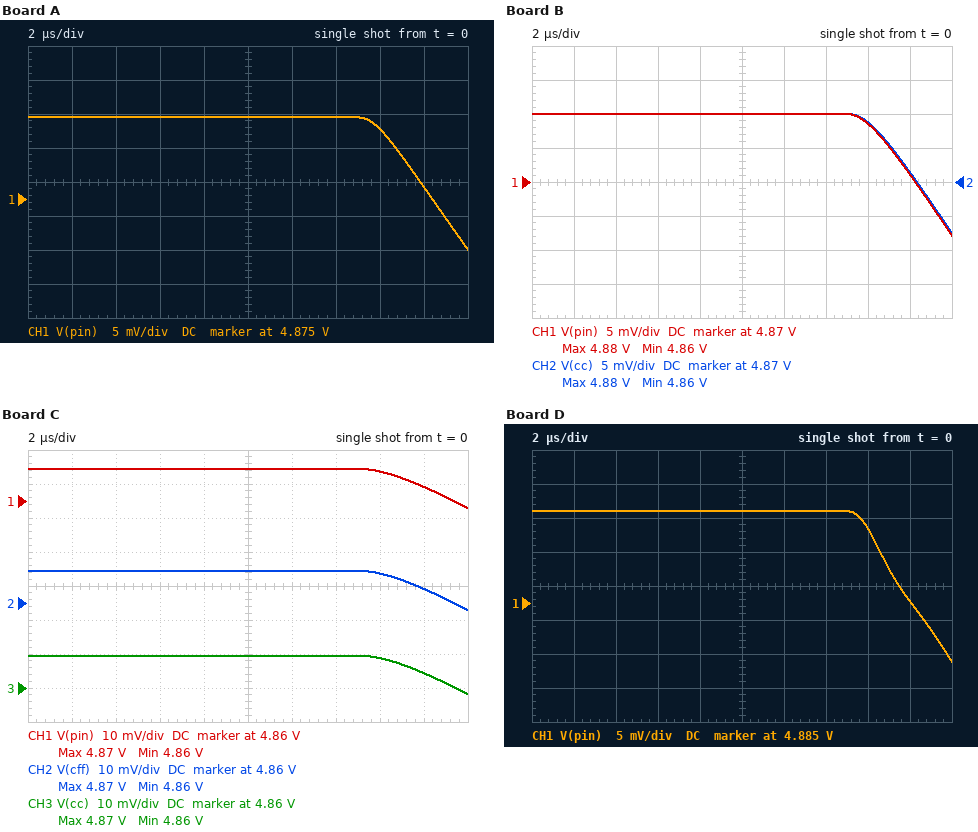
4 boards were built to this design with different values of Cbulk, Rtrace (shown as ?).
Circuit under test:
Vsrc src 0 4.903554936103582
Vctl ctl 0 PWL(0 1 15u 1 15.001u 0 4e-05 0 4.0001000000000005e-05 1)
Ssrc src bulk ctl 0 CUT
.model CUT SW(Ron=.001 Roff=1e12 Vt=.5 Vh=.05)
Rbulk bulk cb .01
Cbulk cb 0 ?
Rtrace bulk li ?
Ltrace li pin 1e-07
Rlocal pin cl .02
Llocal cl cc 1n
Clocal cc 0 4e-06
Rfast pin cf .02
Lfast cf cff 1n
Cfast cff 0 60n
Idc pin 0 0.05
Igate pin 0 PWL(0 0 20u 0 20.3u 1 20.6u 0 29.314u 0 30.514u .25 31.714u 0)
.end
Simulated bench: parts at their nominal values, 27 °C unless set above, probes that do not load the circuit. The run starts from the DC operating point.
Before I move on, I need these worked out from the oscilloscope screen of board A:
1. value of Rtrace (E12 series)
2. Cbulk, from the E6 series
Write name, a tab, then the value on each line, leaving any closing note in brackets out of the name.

value of Rtrace	0.33 Ω
Cbulk, from the E6 series	6.8 µF
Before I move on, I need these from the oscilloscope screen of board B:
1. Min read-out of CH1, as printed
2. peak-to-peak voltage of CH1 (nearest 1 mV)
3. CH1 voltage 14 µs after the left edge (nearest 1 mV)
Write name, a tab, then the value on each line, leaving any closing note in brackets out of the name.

Min read-out of CH1, as printed	4.86 V
peak-to-peak voltage of CH1	18 mV
CH1 voltage 14 µs after the left edge	4.880 V
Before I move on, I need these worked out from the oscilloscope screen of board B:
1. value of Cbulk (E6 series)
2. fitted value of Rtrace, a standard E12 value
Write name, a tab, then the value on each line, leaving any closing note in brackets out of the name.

value of Cbulk	6.8 µF
fitted value of Rtrace, a standard E12 value	0.47 Ω
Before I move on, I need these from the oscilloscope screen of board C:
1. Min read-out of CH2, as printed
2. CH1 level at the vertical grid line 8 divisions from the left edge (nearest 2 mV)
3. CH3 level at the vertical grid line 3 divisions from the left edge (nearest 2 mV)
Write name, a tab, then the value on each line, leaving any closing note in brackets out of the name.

Min read-out of CH2, as printed	4.86 V
CH1 level at the vertical grid line 8 divisions from the left edge	4.868 V
CH3 level at the vertical grid line 3 divisions from the left edge	4.870 V
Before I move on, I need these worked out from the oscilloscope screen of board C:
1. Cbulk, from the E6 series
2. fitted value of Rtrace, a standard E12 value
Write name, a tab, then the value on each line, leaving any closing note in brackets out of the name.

Cbulk, from the E6 series	10 µF
fitted value of Rtrace, a standard E12 value	0.68 Ω
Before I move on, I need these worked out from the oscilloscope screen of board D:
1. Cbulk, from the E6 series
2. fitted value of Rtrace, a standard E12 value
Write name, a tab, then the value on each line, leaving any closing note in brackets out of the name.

Cbulk, from the E6 series	6.8 µF
fitted value of Rtrace, a standard E12 value	0.1 Ω
